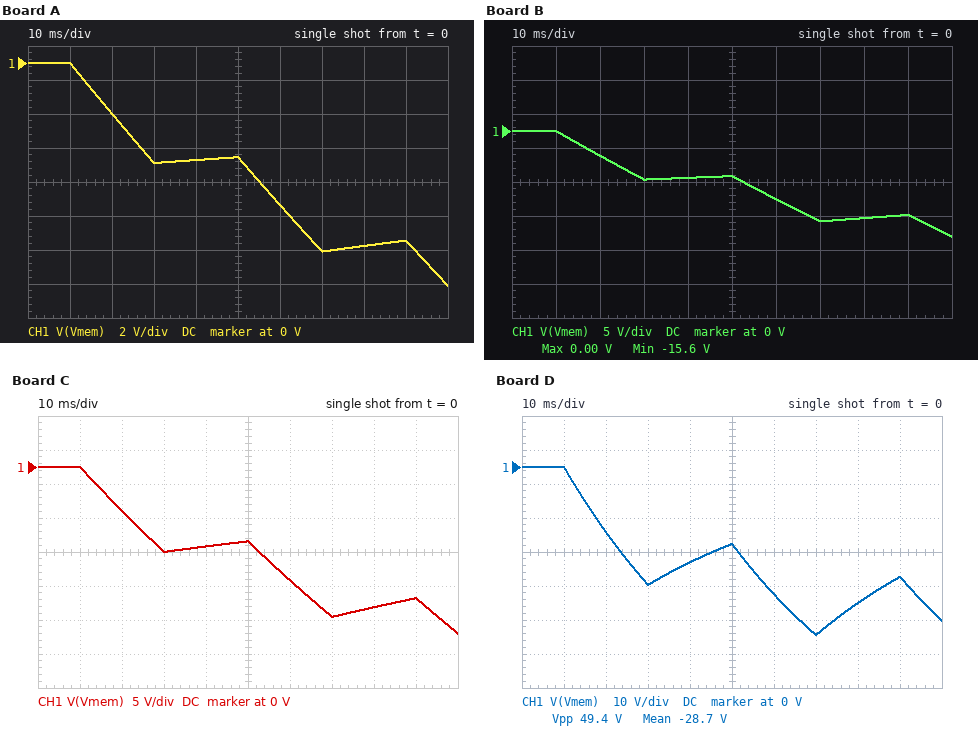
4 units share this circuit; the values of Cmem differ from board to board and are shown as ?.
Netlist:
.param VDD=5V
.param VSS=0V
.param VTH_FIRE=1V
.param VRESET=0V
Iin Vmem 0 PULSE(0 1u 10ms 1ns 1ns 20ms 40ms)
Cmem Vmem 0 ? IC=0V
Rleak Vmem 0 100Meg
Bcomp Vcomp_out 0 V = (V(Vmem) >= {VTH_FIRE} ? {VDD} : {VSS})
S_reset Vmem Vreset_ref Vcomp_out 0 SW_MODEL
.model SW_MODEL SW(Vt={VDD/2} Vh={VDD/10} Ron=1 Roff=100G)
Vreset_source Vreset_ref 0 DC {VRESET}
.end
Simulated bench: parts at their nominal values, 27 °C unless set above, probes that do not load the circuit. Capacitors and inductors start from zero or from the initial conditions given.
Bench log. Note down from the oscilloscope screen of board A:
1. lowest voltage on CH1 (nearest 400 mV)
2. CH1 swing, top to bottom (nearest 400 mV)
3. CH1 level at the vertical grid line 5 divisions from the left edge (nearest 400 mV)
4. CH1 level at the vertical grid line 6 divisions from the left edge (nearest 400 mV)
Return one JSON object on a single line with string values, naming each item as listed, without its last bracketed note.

{"lowest voltage on CH1": "-13.2 V", "CH1 swing, top to bottom": "13.2 V", "CH1 level at the vertical grid line 5 divisions from the left edge": "-5.6 V", "CH1 level at the vertical grid line 6 divisions from the left edge": "-8.4 V"}
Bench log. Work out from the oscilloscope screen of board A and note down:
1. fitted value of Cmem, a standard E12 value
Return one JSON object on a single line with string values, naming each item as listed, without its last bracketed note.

{"fitted value of Cmem, a standard E12 value": "3.3 nF"}
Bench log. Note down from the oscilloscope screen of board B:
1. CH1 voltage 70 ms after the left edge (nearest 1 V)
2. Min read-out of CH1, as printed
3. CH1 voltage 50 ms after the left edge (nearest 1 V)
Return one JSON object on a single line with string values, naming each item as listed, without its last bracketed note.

{"CH1 voltage 70 ms after the left edge": "-13 V", "Min read-out of CH1, as printed": "-15.6 V", "CH1 voltage 50 ms after the left edge": "-7 V"}
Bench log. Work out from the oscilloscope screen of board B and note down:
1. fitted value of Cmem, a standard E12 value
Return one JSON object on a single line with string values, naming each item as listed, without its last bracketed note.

{"fitted value of Cmem, a standard E12 value": "2.7 nF"}
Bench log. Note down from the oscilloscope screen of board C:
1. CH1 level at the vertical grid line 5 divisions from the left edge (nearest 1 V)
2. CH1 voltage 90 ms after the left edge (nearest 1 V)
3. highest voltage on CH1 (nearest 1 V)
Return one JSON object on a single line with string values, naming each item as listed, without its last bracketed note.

{"CH1 level at the vertical grid line 5 divisions from the left edge": "-11 V", "CH1 voltage 90 ms after the left edge": "-19 V", "highest voltage on CH1": "0 V"}
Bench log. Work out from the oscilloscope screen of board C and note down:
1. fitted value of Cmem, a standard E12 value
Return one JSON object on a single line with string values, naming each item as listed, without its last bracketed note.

{"fitted value of Cmem, a standard E12 value": "1.5 nF"}
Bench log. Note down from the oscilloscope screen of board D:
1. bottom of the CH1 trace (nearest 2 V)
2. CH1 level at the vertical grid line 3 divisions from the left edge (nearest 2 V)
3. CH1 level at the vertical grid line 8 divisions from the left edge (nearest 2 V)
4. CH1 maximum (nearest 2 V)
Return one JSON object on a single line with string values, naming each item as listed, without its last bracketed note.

{"bottom of the CH1 trace": "-50 V", "CH1 level at the vertical grid line 3 divisions from the left edge": "-34 V", "CH1 level at the vertical grid line 8 divisions from the left edge": "-40 V", "CH1 maximum": "0 V"}
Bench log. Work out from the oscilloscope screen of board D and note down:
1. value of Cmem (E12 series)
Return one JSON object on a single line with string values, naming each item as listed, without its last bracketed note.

{"value of Cmem": "470 pF"}
